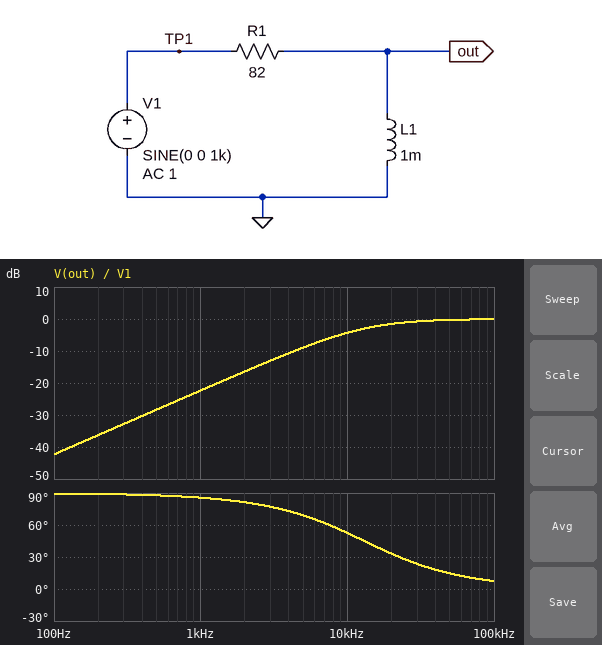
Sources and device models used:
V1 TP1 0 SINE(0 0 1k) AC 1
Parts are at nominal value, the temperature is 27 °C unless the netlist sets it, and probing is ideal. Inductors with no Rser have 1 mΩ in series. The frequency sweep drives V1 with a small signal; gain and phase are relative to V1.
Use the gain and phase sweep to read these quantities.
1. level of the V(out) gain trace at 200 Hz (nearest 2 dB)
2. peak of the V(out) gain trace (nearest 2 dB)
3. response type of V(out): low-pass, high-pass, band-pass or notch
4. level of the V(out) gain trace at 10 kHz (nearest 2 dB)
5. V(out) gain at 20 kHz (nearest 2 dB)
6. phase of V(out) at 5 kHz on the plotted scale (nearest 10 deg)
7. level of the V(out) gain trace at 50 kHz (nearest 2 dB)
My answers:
-36 dB
0 dB
high-pass
-4 dB
-2 dB
70 deg
0 dB
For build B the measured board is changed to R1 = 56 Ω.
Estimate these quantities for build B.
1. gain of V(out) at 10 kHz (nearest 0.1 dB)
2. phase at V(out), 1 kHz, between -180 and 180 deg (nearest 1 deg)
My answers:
-2.5 dB
84 deg
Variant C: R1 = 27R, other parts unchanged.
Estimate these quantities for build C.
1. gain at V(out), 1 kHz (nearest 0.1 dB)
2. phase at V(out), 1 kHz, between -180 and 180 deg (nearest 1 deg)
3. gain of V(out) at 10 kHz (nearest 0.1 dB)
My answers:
-12.9 dB
77 deg
-0.7 dB
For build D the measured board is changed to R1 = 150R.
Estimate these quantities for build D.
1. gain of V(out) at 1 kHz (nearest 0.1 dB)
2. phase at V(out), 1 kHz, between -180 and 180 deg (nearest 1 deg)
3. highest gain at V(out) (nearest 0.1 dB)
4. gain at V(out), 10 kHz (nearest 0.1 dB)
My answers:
-27.6 dB
88 deg
0 dB
-8.3 dB
